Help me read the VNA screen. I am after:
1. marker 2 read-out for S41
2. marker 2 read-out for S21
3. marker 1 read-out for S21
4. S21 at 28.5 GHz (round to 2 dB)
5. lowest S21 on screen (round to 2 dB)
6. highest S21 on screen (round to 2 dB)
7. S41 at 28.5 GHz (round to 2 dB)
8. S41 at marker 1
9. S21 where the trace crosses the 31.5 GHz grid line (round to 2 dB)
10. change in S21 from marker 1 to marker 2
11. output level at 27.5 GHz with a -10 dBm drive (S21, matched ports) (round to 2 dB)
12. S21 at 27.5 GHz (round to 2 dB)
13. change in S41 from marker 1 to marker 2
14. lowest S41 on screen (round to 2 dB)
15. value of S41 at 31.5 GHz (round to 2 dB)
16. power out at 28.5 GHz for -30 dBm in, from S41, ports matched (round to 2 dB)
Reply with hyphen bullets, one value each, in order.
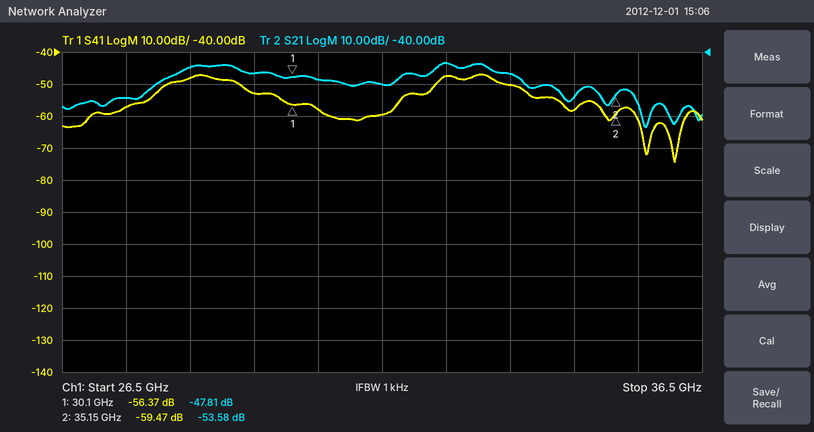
- -59.47 dB
- -53.58 dB
- -47.81 dB
- -44 dB
- -64 dB
- -44 dB
- -48 dB
- -56.37 dB
- -50 dB
- -5.77 dB
- -64 dBm
- -54 dB
- -3.10 dB
- -74 dB
- -60 dB
- -78 dBm
